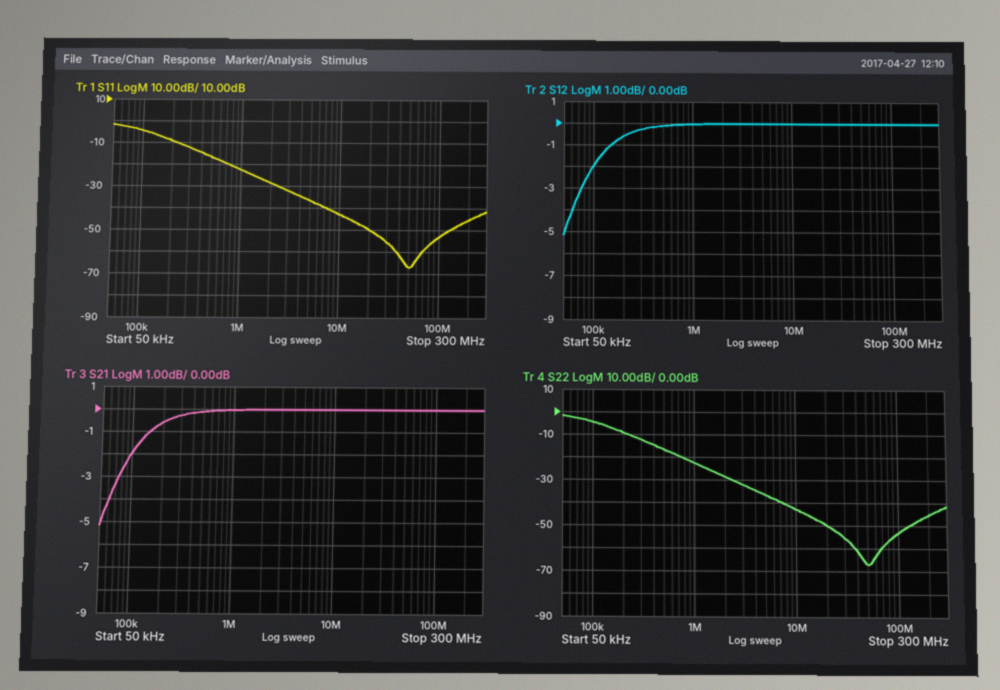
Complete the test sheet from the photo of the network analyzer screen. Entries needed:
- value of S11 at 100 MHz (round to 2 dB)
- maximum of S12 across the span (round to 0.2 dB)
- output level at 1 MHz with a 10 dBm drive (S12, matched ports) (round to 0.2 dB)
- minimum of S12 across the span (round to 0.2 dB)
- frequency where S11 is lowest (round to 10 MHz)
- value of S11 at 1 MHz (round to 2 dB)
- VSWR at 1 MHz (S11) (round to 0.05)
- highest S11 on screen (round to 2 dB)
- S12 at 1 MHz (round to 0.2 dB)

-54 dB
0.0 dB
10.0 dBm
-5.2 dB
50 MHz
-22 dB
1.15
-2 dB
0.0 dB
